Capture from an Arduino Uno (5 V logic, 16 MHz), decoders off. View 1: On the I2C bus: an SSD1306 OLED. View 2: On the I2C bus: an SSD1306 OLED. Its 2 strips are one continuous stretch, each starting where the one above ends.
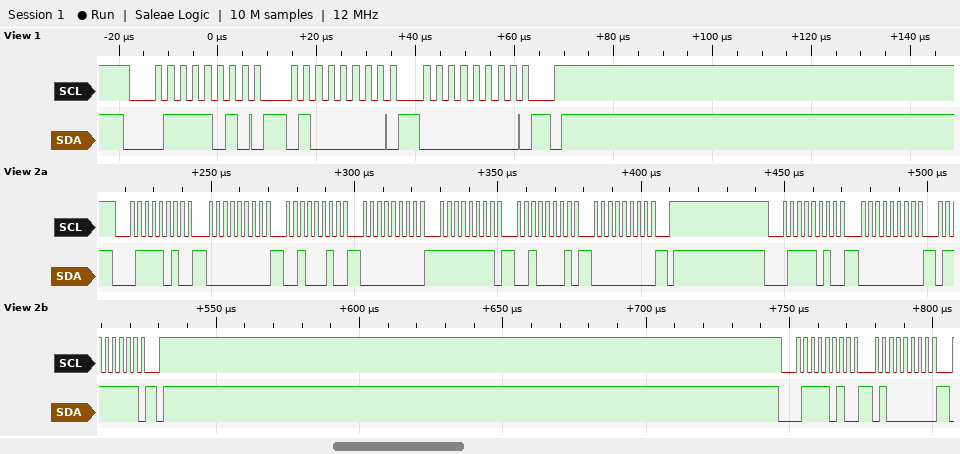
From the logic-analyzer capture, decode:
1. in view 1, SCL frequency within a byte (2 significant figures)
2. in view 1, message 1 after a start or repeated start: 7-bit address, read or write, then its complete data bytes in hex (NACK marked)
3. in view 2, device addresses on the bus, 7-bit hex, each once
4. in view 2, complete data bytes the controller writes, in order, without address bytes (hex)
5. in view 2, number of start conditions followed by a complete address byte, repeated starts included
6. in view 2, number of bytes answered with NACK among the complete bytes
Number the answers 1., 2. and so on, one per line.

1. 400 kHz
2. 0x3D write: 40 00
3. 0x3D
4. 00 22 00 FF 21 00 00 7F 40
5. 3
6. 0
